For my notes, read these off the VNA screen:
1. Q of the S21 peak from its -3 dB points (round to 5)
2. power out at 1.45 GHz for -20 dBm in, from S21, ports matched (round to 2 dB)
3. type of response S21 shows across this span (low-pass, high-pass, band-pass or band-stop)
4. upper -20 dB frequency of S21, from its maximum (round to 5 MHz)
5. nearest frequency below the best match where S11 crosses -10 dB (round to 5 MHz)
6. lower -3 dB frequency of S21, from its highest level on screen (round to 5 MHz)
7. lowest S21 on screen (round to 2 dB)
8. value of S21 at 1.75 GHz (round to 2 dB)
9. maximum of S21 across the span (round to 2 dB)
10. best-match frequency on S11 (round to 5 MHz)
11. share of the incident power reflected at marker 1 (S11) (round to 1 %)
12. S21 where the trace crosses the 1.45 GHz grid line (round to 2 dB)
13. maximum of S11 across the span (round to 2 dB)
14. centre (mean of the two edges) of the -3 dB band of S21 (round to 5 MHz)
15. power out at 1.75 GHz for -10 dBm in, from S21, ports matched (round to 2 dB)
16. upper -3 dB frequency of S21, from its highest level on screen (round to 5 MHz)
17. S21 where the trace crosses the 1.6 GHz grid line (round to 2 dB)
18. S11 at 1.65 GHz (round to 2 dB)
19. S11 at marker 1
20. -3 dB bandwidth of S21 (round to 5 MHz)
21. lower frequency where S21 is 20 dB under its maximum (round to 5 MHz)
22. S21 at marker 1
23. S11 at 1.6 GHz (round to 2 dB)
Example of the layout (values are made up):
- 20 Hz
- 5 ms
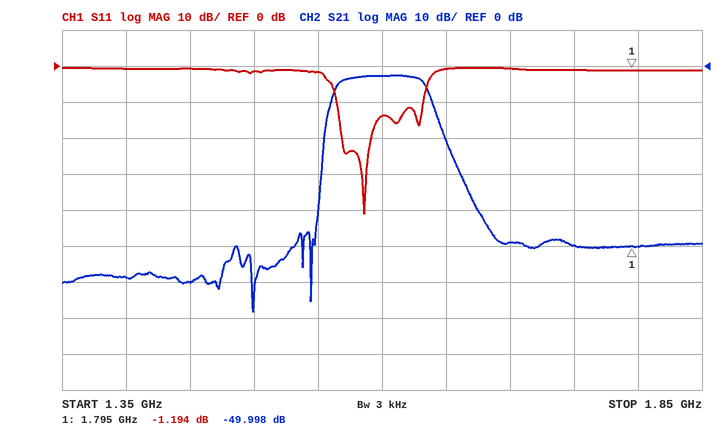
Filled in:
- 25
- -80 dBm
- band-pass
- 1.650 GHz
- 1.565 GHz
- 1.565 GHz
- -68 dB
- -50 dB
- -2 dB
- 1.585 GHz
- 76 %
- -60 dB
- 0 dB
- 1.600 GHz
- -60 dBm
- 1.635 GHz
- -2 dB
- 0 dB
- -1.194 dB
- 70 MHz
- 1.555 GHz
- -49.998 dB
- -14 dB
